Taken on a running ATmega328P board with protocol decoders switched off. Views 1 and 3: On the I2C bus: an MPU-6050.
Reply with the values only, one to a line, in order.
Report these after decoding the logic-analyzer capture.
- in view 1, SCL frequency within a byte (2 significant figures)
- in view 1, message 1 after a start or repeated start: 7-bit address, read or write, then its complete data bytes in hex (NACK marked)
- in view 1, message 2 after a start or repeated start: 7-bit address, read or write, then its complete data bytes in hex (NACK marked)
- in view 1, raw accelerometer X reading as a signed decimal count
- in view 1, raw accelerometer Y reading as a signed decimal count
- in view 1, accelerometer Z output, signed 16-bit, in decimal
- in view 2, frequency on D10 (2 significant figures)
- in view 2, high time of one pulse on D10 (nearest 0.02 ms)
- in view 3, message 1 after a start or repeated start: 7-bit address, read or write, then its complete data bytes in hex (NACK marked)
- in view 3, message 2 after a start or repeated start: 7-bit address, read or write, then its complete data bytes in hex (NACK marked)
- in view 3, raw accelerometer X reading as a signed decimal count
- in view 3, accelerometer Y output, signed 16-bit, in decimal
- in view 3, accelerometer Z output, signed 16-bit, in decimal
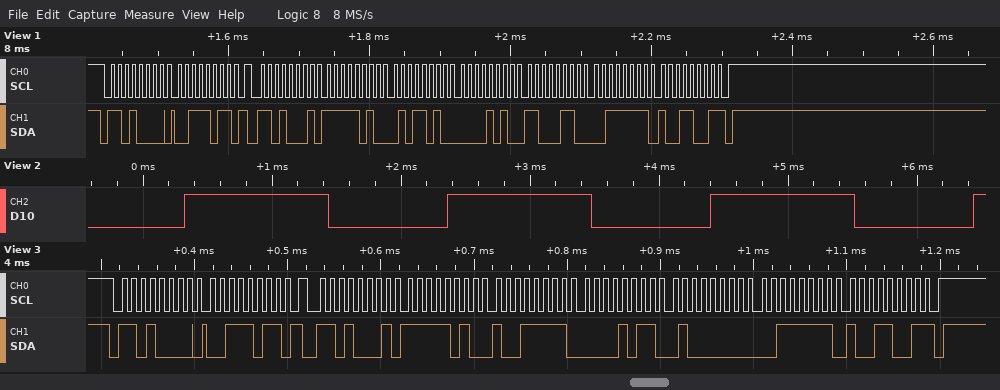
100 kHz
0x68 write: 3B
0x68 read: FA 5A 0A C6 3F 99 NACK
-1446
2758
16281
490 Hz
1.12 ms
0x68 write: 3B
0x68 read: FA 9F 0B 40 3F 99 NACK
-1377
2880
16281
